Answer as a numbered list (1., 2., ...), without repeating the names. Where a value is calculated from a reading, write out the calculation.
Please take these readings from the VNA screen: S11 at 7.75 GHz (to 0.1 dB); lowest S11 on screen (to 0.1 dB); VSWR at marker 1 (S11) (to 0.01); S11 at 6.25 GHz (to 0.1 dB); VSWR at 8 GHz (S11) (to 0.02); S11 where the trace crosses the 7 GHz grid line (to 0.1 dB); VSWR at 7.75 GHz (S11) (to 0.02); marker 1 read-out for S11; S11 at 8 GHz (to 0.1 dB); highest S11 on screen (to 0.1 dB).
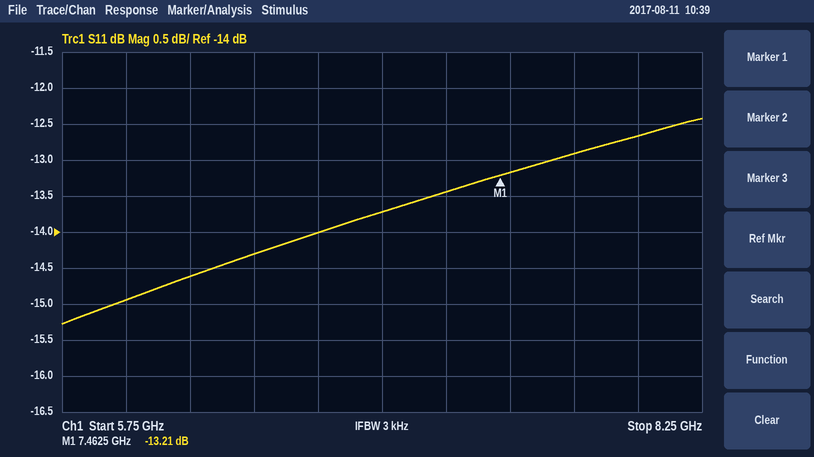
1. -12.9 dB
2. -15.3 dB
3. (1 + 0.2185)/(1 − 0.2185) ≈ 1.56
4. -14.6 dB
5. |Γ| = 10^(-12.7/20) = 0.2317; VSWR = (1 + 0.2317)/(1 − 0.2317) ≈ 1.60
6. -13.7 dB
7. |Γ| = 10^(-12.9/20) = 0.2265; VSWR = (1 + 0.2265)/(1 − 0.2265) ≈ 1.59, so 1.58 to the nearest 0.02
8. -13.21 dB
9. -12.7 dB
10. -12.4 dB
